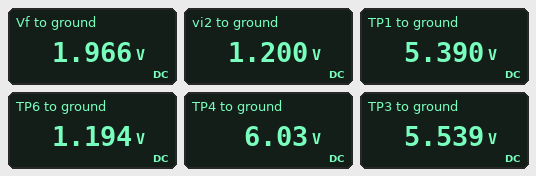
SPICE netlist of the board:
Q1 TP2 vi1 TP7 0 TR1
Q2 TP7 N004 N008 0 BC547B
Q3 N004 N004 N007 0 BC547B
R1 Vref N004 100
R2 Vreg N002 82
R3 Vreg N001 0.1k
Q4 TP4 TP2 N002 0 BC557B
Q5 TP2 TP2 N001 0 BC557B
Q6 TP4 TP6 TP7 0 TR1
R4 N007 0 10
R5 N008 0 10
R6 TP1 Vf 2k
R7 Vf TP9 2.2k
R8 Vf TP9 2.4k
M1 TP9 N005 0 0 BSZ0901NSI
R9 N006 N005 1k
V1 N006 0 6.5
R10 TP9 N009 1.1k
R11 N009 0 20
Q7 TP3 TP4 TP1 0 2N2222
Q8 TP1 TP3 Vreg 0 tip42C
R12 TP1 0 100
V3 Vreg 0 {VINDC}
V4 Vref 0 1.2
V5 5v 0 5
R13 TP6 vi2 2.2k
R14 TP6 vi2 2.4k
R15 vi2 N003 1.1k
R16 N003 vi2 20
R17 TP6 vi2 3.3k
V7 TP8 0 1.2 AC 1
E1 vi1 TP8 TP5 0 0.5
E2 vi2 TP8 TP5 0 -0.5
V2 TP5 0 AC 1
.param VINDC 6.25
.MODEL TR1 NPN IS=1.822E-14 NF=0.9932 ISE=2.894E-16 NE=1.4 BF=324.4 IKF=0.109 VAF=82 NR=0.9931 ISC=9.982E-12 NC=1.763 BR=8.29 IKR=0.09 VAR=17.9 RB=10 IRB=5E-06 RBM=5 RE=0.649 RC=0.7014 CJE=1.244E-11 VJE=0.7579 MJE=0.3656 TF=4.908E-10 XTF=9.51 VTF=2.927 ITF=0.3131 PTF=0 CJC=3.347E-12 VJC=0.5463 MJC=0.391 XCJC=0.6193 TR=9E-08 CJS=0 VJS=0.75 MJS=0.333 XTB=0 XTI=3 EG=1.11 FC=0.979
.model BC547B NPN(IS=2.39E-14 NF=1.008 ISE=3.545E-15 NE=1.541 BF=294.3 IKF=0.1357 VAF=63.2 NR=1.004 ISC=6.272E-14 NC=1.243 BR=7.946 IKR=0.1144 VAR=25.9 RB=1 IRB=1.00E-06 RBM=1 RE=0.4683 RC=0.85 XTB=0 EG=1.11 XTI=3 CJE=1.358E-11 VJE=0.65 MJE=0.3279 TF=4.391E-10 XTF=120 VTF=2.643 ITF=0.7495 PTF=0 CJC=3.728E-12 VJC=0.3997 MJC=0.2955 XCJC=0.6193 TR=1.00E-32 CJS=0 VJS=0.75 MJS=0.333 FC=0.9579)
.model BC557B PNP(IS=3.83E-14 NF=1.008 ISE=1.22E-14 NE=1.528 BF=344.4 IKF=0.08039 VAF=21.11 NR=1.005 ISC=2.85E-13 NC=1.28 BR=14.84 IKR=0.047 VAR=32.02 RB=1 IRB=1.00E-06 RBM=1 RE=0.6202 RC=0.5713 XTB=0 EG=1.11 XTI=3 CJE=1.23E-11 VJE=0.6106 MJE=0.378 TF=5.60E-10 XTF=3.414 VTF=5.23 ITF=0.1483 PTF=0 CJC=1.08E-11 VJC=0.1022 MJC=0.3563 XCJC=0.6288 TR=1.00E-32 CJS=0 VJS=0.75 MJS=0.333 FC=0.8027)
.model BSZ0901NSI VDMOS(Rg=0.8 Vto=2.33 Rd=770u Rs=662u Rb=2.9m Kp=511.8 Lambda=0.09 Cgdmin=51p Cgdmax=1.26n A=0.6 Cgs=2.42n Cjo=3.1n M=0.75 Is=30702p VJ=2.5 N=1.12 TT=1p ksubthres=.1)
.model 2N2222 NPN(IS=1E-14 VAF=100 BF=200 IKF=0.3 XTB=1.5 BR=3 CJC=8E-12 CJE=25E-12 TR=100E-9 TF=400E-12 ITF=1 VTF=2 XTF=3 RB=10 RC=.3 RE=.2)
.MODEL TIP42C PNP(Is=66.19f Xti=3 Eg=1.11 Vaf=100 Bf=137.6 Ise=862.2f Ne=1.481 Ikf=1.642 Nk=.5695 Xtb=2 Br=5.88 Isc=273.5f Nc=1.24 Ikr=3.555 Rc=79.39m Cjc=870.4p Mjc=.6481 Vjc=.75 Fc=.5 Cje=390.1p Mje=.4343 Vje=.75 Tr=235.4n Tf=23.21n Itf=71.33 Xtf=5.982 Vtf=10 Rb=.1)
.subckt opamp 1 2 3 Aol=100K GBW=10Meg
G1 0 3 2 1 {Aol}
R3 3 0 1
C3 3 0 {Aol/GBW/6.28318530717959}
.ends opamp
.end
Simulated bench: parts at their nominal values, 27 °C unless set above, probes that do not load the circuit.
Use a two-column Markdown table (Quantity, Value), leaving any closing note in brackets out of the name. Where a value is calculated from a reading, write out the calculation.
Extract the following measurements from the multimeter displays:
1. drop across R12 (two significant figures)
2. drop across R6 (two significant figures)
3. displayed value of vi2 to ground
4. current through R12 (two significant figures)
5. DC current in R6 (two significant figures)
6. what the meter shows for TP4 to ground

| Quantity | Value |
|---|---|
| drop across R12 | 5.39 V = 5.4 V |
| drop across R6 | 5.39 V - 1.966 V = 3.4 V |
| displayed value of vi2 to ground | 1.200 V |
| current through R12 | (5.39 V) / 100 Ω = 54 mA |
| DC current in R6 | (5.39 V - 1.966 V) / 2 kΩ = 1.7 mA |
| what the meter shows for TP4 to ground | 6.03 V |
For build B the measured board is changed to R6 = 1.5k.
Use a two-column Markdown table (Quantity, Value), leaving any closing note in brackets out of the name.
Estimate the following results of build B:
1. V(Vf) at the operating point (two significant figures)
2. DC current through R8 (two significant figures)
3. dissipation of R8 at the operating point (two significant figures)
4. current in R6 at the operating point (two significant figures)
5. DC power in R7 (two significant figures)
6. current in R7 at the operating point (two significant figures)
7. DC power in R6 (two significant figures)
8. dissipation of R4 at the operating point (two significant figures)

| Quantity | Value |
|---|---|
| V(Vf) at the operating point | 2.3 V |
| DC current through R8 | 970 µA |
| dissipation of R8 at the operating point | 2.3 mW |
| current in R6 at the operating point | 2.0 mA |
| DC power in R7 | 2.5 mW |
| current in R7 at the operating point | 1.1 mA |
| DC power in R6 | 6.2 mW |
| dissipation of R4 at the operating point | 220 µW |
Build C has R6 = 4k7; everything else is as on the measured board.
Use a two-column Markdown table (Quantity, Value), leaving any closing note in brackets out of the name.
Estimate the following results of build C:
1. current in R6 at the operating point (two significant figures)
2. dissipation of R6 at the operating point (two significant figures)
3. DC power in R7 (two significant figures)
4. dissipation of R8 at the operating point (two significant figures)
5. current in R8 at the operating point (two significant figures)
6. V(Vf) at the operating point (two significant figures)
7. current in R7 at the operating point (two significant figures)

| Quantity | Value |
|---|---|
| current in R6 at the operating point | 920 µA |
| dissipation of R6 at the operating point | 4.0 mW |
| DC power in R7 | 510 µW |
| dissipation of R8 at the operating point | 470 µW |
| current in R8 at the operating point | 440 µA |
| V(Vf) at the operating point | 1.1 V |
| current in R7 at the operating point | 480 µA |
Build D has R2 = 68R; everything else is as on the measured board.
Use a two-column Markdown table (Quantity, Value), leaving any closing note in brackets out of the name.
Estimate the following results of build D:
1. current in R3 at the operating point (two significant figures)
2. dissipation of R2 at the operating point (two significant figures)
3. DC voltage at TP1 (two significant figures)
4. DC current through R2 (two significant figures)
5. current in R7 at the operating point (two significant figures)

| Quantity | Value |
|---|---|
| current in R3 at the operating point | 2.1 mA |
| dissipation of R2 at the operating point | 450 µW |
| DC voltage at TP1 | 5.4 V |
| DC current through R2 | 2.6 mA |
| current in R7 at the operating point | 900 µA |
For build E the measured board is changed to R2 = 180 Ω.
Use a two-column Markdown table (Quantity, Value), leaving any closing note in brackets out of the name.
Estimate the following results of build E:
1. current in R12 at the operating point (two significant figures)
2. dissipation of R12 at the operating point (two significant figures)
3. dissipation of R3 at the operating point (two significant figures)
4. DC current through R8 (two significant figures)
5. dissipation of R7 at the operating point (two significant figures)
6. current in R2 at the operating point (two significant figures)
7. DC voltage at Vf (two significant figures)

| Quantity | Value |
|---|---|
| current in R12 at the operating point | 900 µA |
| dissipation of R12 at the operating point | 81 µW |
| dissipation of R3 at the operating point | 850 µW |
| DC current through R8 | 14 µA |
| dissipation of R7 at the operating point | 490 nW |
| current in R2 at the operating point | 1.7 mA |
| DC voltage at Vf | 33 mV |
